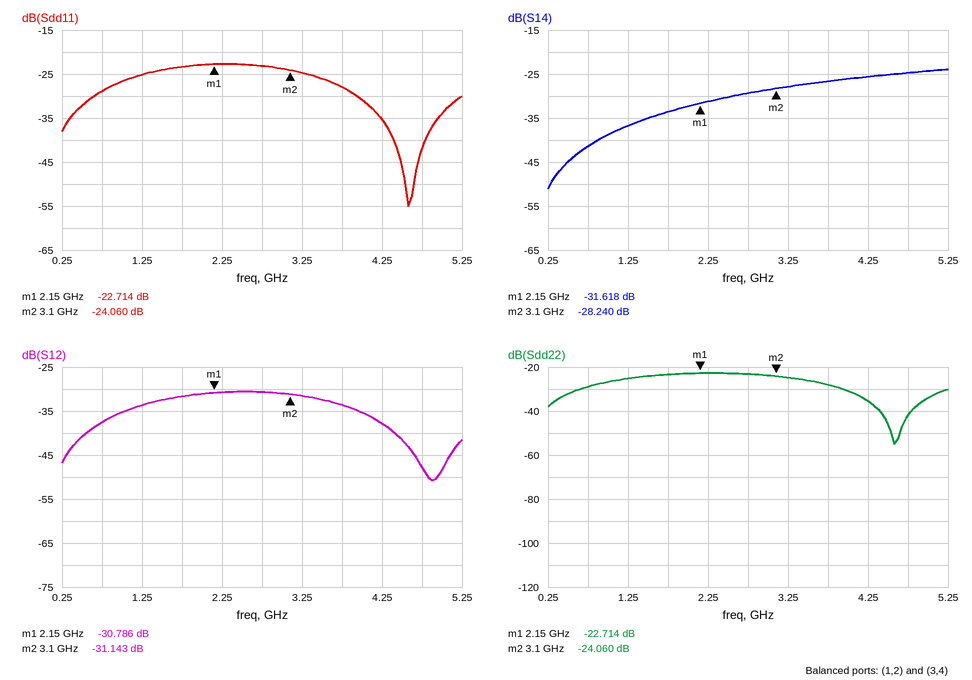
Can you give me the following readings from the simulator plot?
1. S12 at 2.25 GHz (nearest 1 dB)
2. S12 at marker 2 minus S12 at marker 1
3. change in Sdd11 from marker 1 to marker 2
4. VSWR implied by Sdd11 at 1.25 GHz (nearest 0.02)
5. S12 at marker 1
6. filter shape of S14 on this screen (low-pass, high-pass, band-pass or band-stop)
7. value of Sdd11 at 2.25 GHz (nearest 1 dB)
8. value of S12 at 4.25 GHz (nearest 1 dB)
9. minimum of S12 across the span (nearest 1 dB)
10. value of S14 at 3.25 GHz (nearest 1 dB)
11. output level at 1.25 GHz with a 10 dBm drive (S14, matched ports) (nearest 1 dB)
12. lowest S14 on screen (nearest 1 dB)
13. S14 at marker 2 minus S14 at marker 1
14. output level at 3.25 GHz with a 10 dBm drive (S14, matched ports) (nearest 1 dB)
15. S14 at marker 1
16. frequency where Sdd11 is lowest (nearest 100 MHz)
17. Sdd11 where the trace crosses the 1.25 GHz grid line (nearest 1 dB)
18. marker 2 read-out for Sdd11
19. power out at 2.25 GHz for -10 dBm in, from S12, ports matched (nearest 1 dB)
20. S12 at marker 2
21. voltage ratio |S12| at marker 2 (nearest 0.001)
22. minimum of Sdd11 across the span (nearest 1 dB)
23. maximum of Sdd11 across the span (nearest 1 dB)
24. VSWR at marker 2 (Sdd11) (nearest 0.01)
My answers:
-31 dB
-0.357 dB
-1.346 dB
1.12
-30.786 dB
high-pass
-23 dB
-38 dB
-51 dB
-28 dB
-27 dBm
-51 dB
3.378 dB
-18 dBm
-31.618 dB
4.6 GHz
-25 dB
-24.060 dB
-41 dBm
-31.143 dB
0.028
-55 dB
-23 dB
1.13
